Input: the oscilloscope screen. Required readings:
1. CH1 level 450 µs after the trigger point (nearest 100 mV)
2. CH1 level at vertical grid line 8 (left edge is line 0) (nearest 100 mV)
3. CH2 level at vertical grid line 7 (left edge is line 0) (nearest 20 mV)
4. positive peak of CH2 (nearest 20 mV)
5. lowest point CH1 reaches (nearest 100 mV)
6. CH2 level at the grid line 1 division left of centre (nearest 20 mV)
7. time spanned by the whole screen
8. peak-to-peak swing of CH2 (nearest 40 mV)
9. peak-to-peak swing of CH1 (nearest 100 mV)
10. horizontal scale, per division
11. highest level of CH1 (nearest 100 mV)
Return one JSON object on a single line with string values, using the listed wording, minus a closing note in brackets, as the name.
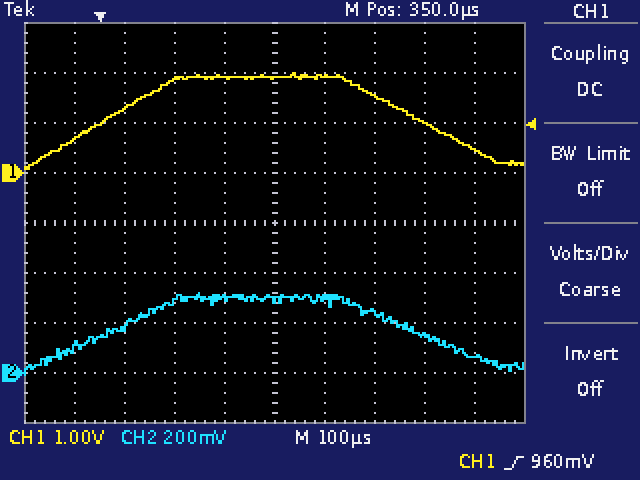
{"CH1 level 450 µs after the trigger point": "1.9 V", "CH1 level at vertical grid line 8 (left edge is line 0)": "1.0 V", "CH2 level at vertical grid line 7 (left edge is line 0)": "240 mV", "positive peak of CH2": "320 mV", "lowest point CH1 reaches": "100 mV", "CH2 level at the grid line 1 division left of centre": "300 mV", "time spanned by the whole screen": "1 ms", "peak-to-peak swing of CH2": "320 mV", "peak-to-peak swing of CH1": "1.9 V", "horizontal scale, per division": "100 µs", "highest level of CH1": "2.0 V"}
